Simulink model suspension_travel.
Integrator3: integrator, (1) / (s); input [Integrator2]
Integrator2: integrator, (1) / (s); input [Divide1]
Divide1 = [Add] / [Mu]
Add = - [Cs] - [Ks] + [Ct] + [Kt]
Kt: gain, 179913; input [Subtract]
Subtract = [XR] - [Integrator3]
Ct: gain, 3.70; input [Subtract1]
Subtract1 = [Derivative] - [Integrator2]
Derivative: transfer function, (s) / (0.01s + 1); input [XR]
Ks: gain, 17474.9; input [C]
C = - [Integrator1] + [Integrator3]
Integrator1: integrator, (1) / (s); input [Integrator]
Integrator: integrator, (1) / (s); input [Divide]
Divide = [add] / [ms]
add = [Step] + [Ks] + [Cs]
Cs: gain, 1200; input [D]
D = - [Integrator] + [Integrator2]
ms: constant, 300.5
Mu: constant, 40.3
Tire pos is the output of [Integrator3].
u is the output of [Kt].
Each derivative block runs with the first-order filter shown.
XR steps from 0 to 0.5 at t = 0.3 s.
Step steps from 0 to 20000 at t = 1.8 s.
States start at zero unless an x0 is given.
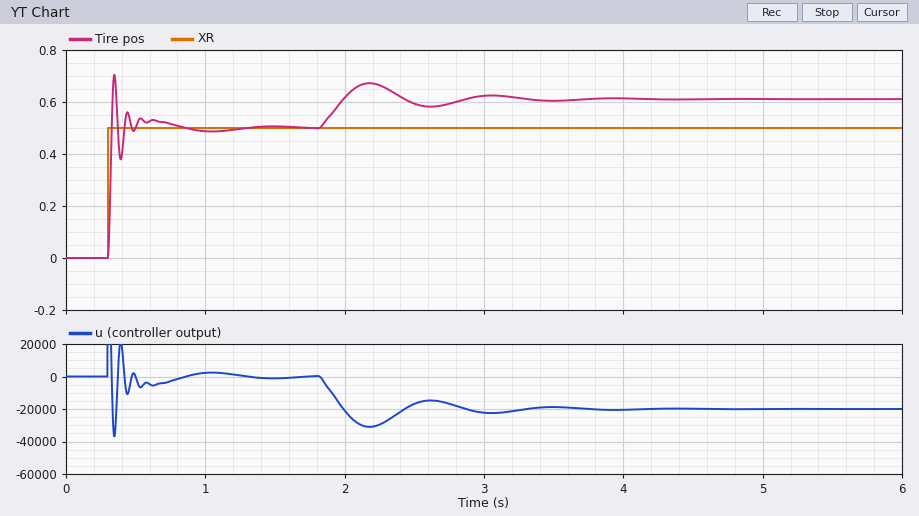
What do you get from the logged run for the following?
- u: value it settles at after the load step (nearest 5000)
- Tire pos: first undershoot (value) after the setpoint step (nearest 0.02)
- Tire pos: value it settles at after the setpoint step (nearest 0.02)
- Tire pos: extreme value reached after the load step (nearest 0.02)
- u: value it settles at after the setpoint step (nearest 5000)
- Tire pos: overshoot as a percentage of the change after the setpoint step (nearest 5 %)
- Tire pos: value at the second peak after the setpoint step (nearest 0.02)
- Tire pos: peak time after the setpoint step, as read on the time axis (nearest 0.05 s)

-20000
0.38
0.50
0.68
0
40 %
0.56
0.35 s
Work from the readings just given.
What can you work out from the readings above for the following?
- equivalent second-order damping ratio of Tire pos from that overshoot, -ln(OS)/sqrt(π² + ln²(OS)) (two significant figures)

0.28
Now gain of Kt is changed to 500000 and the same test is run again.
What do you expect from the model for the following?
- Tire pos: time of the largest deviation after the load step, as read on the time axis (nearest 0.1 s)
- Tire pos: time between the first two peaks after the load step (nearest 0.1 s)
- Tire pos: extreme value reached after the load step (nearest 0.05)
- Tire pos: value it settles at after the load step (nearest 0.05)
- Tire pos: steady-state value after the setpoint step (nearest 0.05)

2.2 s
0.9 s
0.55
0.55
0.50
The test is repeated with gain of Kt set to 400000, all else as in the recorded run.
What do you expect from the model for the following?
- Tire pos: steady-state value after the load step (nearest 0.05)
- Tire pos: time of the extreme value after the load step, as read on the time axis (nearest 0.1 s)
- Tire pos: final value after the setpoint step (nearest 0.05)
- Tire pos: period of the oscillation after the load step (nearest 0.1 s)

0.55
2.2 s
0.50
0.9 s
